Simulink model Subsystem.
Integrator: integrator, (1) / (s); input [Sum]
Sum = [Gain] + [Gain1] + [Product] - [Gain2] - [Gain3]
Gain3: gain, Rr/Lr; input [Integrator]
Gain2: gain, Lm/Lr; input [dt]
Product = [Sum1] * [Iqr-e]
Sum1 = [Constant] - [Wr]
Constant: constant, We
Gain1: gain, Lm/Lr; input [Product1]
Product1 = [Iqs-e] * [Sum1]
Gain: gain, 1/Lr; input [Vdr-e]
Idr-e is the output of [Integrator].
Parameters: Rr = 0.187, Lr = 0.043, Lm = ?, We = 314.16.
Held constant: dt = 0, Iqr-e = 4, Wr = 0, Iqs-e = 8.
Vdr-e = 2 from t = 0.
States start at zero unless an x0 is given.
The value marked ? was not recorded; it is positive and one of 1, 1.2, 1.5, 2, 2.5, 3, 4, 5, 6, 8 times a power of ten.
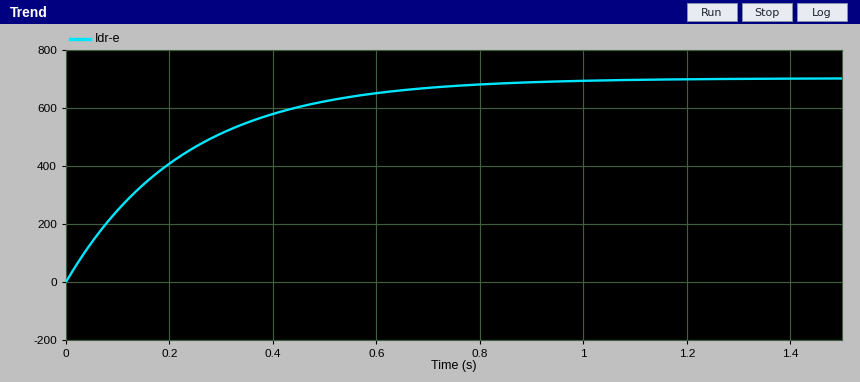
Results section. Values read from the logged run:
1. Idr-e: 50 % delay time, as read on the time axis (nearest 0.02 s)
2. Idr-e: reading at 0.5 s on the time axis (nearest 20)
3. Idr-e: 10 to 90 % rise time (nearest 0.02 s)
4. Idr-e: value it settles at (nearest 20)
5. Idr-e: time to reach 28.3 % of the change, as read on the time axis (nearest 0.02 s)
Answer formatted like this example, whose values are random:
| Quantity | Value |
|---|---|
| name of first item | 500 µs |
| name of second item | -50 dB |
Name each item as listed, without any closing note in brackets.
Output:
| Quantity | Value |
|---|---|
| Idr-e: 50 % delay time, as read on the time axis | 0.16 s |
| Idr-e: reading at 0.5 s on the time axis | 620 |
| Idr-e: 10 to 90 % rise time | 0.50 s |
| Idr-e: value it settles at | 700 |
| Idr-e: time to reach 28.3 % of the change, as read on the time axis | 0.08 s |
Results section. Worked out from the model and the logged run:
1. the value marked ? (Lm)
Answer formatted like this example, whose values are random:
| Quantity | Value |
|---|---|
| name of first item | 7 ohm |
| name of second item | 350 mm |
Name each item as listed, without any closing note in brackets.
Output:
| Quantity | Value |
|---|---|
| the value marked ? | 0.03 |
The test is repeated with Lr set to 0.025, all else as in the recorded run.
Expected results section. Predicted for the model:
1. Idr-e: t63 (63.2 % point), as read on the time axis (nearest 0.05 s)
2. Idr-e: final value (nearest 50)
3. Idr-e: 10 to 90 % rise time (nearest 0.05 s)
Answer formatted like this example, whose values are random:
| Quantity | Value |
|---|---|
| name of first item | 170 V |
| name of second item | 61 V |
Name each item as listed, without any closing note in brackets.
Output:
| Quantity | Value |
|---|---|
| Idr-e: t63 (63.2 % point), as read on the time axis | 0.15 s |
| Idr-e: final value | 600 |
| Idr-e: 10 to 90 % rise time | 0.30 s |
